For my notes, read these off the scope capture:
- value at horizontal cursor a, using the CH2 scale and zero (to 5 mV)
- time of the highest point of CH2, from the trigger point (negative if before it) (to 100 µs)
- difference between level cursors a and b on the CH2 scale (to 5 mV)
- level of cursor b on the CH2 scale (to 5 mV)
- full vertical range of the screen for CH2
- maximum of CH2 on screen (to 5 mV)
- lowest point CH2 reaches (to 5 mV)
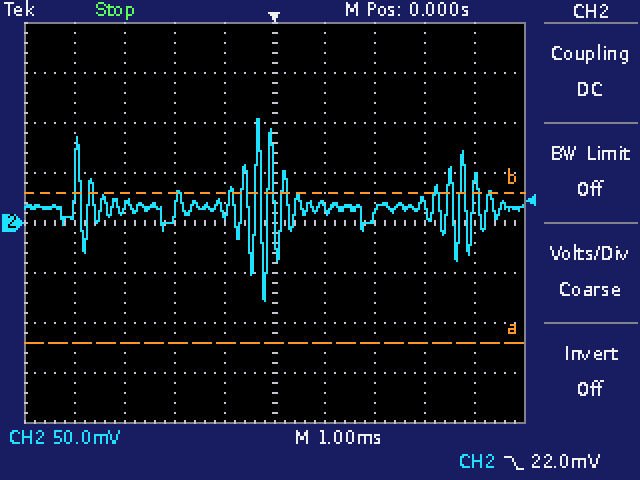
-120 mV
-300 µs
150 mV
30 mV
400 mV
105 mV
-80 mV
